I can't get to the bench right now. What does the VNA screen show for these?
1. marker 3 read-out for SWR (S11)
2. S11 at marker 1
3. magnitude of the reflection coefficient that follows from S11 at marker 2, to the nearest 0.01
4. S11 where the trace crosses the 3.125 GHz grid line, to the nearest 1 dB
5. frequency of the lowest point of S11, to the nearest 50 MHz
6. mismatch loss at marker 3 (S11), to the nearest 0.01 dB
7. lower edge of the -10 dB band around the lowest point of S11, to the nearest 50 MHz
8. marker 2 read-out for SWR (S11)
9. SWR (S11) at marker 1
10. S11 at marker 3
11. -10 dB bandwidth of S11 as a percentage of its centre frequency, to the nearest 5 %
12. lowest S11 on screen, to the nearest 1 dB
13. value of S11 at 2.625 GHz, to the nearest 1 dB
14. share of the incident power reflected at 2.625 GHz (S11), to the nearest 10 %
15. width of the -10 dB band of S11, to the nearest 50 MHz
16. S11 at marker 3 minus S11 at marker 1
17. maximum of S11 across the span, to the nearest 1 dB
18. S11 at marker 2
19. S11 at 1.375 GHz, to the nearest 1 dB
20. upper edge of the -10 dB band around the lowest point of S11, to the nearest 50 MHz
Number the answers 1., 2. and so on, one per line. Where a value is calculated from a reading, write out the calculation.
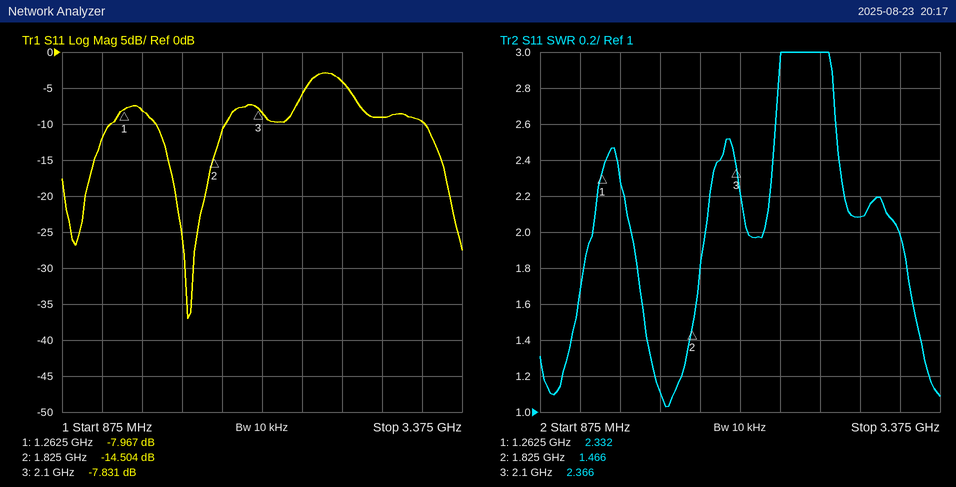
1. 2.366
2. -7.967 dB
3. 10^(-14.504/20) ≈ 0.19
4. -10 dB
5. 1.65 GHz
6. −10 log10(1 − 10^(-7.831/10)) ≈ 0.78 dB
7. 1.45 GHz
8. 1.466
9. 2.332
10. -7.831 dB
11. 450 MHz / 1.675 GHz ≈ 26.9 %, so 25 % to the nearest 5 %
12. -37 dB
13. -4 dB
14. 10^(-4/10) ≈ 40 %
15. 1.90 GHz − 1.45 GHz = 450 MHz
16. -7.831 − (-7.967) = 0.136 dB
17. -3 dB
18. -14.504 dB
19. -8 dB
20. 1.90 GHz
